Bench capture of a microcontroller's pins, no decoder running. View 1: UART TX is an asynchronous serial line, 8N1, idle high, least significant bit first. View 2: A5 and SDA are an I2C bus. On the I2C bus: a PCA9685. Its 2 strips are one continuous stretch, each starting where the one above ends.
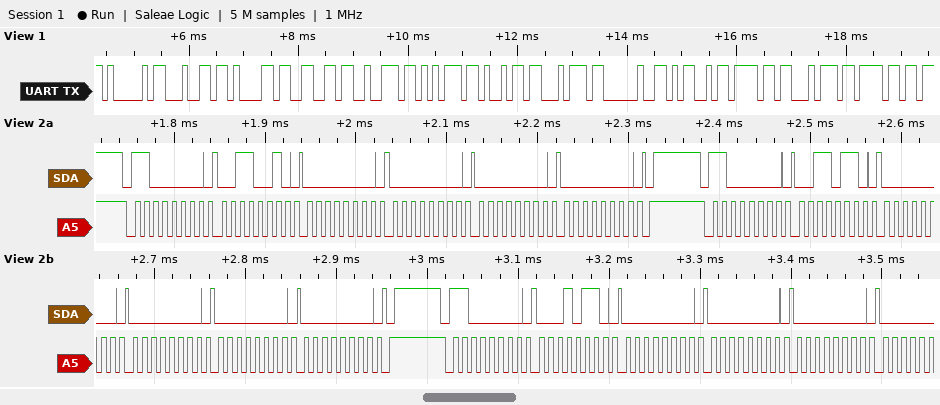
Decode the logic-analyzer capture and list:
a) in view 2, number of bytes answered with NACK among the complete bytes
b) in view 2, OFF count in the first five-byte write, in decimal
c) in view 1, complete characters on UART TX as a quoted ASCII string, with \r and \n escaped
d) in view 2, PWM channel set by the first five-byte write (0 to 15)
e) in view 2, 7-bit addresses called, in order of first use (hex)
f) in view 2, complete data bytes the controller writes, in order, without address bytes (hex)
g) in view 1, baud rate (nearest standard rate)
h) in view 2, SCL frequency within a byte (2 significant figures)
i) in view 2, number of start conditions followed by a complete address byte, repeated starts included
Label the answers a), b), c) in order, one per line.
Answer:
a) 0
b) 0
c) "Adafruit Moto"
d) 11
e) 0x60
f) 32 00 00 00 00 36 00 00 00 00 16 00 00 00
g) 9600 baud
h) 100 kHz
i) 3
